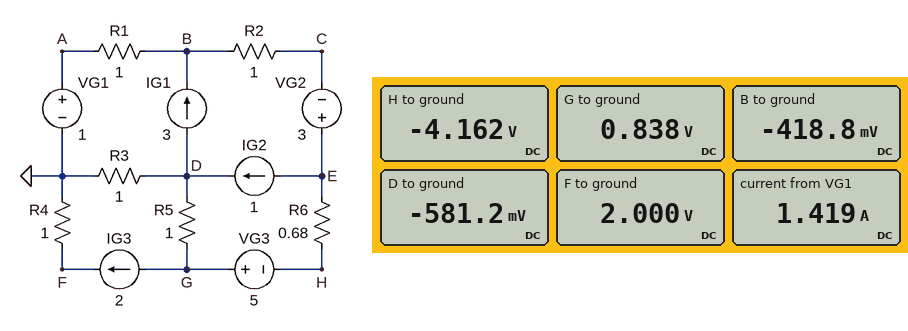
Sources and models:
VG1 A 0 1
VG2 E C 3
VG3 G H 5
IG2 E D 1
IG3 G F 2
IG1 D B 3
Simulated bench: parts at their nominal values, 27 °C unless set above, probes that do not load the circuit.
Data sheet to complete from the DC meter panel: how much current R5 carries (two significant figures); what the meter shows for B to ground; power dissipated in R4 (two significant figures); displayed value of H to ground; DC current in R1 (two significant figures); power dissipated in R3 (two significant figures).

1.4 A
-418.8 mV
4.0 W
-4.162 V
1.4 A
340 mW
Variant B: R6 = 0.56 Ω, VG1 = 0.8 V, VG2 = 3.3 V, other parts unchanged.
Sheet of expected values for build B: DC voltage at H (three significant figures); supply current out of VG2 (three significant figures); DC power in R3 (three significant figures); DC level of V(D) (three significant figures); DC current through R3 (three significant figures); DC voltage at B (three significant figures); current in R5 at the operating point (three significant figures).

-3.94 V
4.53 A
220 mW
-469 mV
469 mA
-731 mV
1.53 A
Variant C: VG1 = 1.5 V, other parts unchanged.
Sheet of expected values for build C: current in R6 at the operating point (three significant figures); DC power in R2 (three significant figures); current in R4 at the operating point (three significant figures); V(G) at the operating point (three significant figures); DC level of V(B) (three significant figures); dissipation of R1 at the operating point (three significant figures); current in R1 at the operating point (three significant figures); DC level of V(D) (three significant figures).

3.53 A
20.5 W
2.00 A
1.05 V
-25.6 mV
2.33 W
1.53 A
-474 mV
